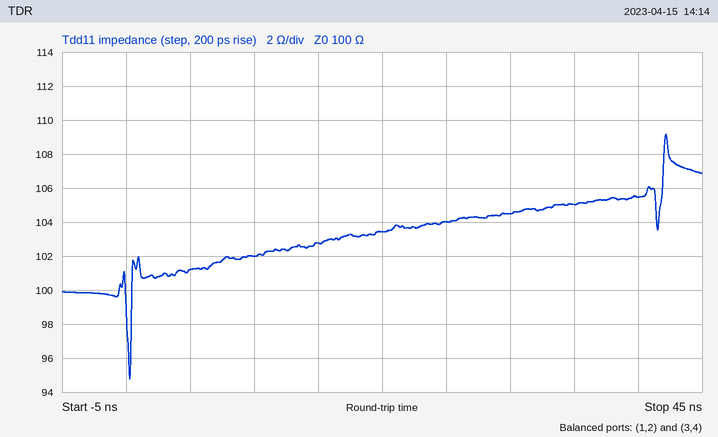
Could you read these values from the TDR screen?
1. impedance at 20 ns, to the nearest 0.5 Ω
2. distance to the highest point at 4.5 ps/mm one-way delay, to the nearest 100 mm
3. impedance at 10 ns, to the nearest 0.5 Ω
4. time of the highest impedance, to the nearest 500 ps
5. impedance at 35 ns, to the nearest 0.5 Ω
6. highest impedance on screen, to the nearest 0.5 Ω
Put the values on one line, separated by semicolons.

103.5 Ω; 4.7 m; 102.0 Ω; 42.0 ns; 105.0 Ω; 109.0 Ω
